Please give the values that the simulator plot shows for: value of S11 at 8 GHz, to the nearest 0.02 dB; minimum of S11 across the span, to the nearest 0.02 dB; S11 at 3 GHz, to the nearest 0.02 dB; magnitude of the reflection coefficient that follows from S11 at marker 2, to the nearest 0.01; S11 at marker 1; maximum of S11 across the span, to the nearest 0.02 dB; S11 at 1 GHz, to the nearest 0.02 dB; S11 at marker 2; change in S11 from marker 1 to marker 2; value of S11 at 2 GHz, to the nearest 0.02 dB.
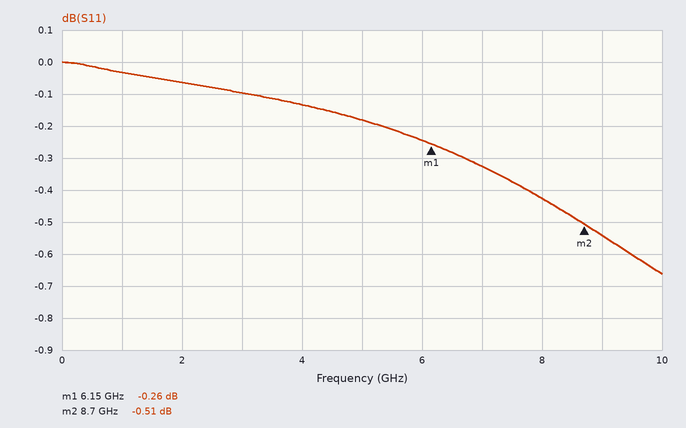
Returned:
-0.42 dB
-0.66 dB
-0.10 dB
0.94
-0.26 dB
0.00 dB
-0.04 dB
-0.51 dB
-0.25 dB
-0.06 dB
